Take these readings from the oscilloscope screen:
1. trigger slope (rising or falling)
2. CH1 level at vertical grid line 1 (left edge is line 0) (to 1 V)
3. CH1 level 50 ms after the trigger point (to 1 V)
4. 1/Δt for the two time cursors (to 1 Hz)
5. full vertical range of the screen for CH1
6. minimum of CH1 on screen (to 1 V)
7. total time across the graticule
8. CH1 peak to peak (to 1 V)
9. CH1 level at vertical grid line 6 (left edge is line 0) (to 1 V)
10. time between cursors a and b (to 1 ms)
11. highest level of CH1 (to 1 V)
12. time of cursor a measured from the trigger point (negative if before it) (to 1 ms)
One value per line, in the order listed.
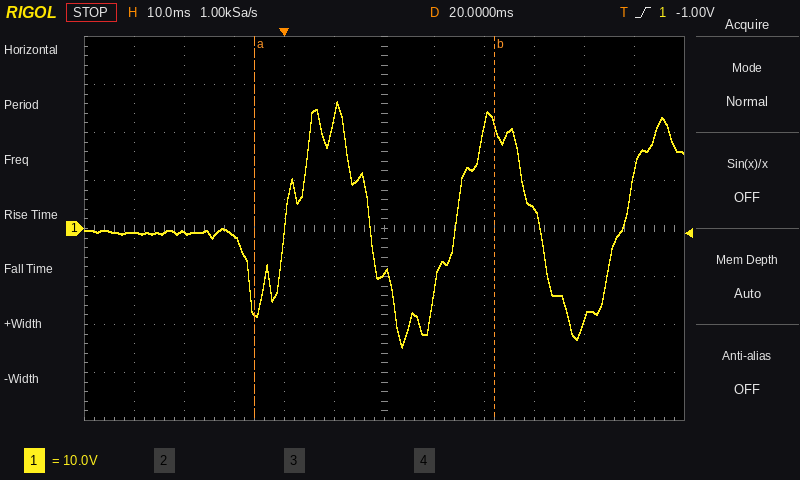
rising
-1 V
4 V
21 Hz
80 V
-25 V
120 ms
51 V
-9 V
48 ms
26 V
-6 ms
